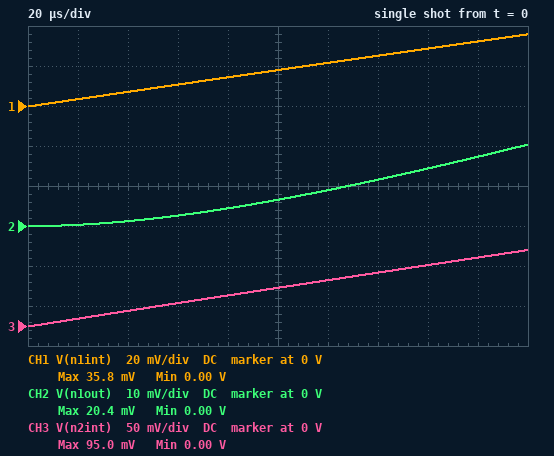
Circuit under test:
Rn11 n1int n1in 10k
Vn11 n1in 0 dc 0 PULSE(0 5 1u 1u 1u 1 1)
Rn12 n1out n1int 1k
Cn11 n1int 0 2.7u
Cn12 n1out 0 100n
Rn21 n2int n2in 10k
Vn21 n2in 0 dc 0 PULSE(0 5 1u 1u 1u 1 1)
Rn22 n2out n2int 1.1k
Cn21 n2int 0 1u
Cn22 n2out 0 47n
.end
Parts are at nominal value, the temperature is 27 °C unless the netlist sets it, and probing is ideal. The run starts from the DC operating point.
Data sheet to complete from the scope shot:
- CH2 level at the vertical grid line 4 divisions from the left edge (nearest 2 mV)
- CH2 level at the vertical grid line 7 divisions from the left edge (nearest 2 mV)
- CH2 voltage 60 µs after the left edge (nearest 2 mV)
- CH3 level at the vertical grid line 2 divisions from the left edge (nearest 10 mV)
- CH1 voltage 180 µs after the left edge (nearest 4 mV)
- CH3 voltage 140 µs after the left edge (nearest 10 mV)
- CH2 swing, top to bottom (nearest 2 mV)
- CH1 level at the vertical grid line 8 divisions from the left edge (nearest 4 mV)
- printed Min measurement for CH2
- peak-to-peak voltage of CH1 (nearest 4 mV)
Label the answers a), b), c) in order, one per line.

a) 4 mV
b) 12 mV
c) 2 mV
d) 20 mV
e) 32 mV
f) 70 mV
g) 20 mV
h) 28 mV
i) 0.00 V
j) 36 mV
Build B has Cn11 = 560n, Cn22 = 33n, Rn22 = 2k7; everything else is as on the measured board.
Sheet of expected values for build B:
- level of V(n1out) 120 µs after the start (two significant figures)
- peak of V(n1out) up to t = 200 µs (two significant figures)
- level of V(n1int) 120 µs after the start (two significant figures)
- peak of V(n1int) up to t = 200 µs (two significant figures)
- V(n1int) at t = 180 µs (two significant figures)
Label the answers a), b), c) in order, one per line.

a) 41 mV
b) 91 mV
c) 97 mV
d) 160 mV
e) 140 mV
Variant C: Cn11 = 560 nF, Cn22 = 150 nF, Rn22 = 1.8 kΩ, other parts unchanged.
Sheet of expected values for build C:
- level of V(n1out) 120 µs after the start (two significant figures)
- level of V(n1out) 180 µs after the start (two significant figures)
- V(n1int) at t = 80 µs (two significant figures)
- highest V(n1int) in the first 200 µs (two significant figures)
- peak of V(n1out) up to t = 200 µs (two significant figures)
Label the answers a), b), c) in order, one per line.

a) 41 mV
b) 78 mV
c) 66 mV
d) 160 mV
e) 91 mV
